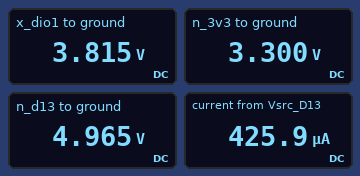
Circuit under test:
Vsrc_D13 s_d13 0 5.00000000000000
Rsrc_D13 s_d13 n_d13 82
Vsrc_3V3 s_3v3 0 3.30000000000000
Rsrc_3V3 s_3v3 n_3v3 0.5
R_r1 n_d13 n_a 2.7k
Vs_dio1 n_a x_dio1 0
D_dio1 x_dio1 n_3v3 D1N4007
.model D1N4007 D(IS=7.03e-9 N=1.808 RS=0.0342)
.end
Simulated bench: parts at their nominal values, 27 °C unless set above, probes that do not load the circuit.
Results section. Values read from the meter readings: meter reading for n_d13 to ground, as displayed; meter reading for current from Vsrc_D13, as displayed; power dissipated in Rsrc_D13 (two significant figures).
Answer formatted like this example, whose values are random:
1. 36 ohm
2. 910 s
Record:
1. 4.965 V
2. 425.9 µA
3. 15 µW
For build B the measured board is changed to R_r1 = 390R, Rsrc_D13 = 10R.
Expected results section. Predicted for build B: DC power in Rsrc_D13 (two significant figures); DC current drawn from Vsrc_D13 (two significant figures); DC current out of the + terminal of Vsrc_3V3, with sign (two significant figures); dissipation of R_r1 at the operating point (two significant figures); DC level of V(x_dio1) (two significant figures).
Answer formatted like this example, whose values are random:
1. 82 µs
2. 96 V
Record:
1. 75 µW
2. 2.7 mA
3. -2.7 mA
4. 2.9 mW
5. 3.9 V
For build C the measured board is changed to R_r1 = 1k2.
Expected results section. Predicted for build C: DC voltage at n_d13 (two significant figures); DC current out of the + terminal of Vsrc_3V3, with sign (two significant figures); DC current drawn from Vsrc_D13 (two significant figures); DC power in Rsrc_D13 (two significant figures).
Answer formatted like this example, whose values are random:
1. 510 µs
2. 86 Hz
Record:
1. 4.9 V
2. -900 µA
3. 900 µA
4. 66 µW
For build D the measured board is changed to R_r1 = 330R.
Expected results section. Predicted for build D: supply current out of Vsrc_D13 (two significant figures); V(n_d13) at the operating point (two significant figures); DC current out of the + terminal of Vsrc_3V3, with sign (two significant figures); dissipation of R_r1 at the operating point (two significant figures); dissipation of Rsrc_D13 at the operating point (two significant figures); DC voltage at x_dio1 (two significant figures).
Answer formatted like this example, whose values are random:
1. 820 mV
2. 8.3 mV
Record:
1. 2.7 mA
2. 4.8 V
3. -2.7 mA
4. 2.3 mW
5. 580 µW
6. 3.9 V
